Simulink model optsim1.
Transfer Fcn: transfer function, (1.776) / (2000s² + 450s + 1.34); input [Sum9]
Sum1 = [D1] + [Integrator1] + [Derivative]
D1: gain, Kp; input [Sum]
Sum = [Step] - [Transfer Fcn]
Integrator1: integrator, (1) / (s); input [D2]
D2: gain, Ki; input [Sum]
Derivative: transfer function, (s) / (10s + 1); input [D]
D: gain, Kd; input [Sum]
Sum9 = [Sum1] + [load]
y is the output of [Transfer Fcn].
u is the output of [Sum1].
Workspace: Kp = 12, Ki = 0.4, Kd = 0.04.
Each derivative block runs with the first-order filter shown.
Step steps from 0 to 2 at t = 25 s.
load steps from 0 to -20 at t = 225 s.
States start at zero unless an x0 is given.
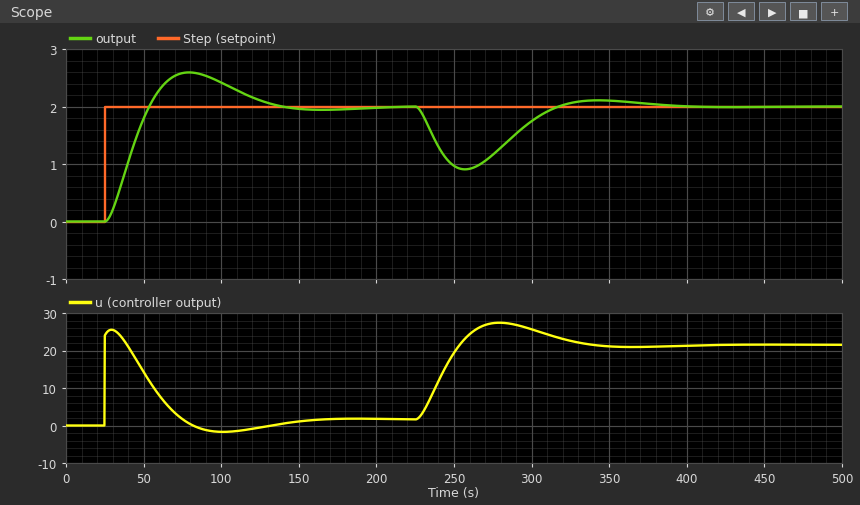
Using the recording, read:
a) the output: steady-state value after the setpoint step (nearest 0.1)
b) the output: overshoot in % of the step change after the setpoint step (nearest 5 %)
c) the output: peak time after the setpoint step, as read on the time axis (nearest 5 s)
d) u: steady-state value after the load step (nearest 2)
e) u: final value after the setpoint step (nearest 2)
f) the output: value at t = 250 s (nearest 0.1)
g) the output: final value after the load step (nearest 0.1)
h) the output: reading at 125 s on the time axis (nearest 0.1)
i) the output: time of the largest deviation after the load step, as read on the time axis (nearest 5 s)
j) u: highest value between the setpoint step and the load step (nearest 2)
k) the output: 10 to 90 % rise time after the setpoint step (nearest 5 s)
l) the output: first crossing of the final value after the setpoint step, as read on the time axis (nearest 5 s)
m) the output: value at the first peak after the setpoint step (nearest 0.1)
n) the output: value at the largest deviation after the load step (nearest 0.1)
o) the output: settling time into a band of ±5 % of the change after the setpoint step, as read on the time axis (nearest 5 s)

2.0
30 %
80 s
22
2
1.0
2.0
2.1
255 s
26
20 s
55 s
2.6
0.9
125 s
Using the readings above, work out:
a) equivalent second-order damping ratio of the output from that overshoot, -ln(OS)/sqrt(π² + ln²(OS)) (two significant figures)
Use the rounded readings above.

0.36
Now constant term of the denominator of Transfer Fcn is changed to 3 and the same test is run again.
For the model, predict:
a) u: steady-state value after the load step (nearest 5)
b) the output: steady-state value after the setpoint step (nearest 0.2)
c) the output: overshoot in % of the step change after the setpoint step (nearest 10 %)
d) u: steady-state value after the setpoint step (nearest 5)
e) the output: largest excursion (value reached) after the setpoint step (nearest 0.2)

25
2.0
20 %
5
2.4
